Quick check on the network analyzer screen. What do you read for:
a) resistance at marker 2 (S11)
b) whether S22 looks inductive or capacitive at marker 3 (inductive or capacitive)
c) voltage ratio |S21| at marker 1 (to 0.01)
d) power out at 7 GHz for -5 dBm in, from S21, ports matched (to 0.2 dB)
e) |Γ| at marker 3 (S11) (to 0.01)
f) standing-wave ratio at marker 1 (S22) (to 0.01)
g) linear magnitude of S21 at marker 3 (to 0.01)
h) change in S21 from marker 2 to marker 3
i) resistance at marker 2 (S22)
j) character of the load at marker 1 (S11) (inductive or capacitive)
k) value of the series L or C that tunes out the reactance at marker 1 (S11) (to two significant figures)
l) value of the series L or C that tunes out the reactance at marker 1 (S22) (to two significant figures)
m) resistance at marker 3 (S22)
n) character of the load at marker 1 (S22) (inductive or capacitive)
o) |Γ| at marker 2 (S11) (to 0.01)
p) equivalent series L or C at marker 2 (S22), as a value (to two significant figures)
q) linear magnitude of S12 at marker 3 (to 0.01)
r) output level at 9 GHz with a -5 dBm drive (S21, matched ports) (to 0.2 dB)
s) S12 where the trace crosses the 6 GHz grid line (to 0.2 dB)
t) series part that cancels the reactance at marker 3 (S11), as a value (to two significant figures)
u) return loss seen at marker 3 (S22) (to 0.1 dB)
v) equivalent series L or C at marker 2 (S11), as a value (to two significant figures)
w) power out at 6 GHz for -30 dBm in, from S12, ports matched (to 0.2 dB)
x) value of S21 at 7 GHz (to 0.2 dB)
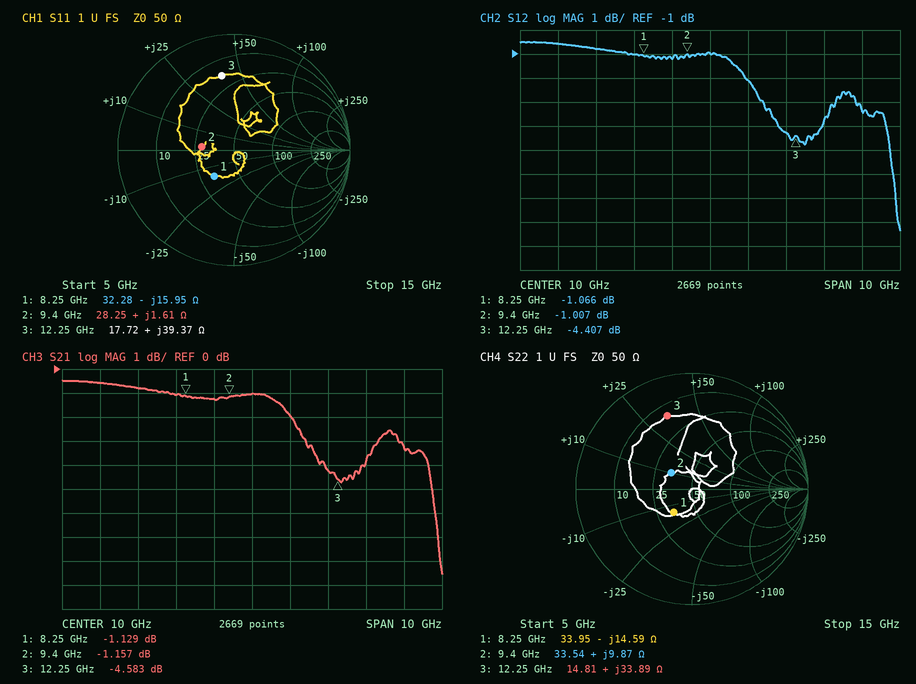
28.25 Ω
inductive
0.88
-5.8 dBm
0.65
1.68
0.59
-3.426 dB
33.54 Ω
capacitive
310 pH
280 pH
14.81 Ω
capacitive
0.28
170 pH
0.60
-6.2 dBm
-0.6 dB
330 fF
3.5 dB
27 pH
-30.6 dBm
-0.8 dB
